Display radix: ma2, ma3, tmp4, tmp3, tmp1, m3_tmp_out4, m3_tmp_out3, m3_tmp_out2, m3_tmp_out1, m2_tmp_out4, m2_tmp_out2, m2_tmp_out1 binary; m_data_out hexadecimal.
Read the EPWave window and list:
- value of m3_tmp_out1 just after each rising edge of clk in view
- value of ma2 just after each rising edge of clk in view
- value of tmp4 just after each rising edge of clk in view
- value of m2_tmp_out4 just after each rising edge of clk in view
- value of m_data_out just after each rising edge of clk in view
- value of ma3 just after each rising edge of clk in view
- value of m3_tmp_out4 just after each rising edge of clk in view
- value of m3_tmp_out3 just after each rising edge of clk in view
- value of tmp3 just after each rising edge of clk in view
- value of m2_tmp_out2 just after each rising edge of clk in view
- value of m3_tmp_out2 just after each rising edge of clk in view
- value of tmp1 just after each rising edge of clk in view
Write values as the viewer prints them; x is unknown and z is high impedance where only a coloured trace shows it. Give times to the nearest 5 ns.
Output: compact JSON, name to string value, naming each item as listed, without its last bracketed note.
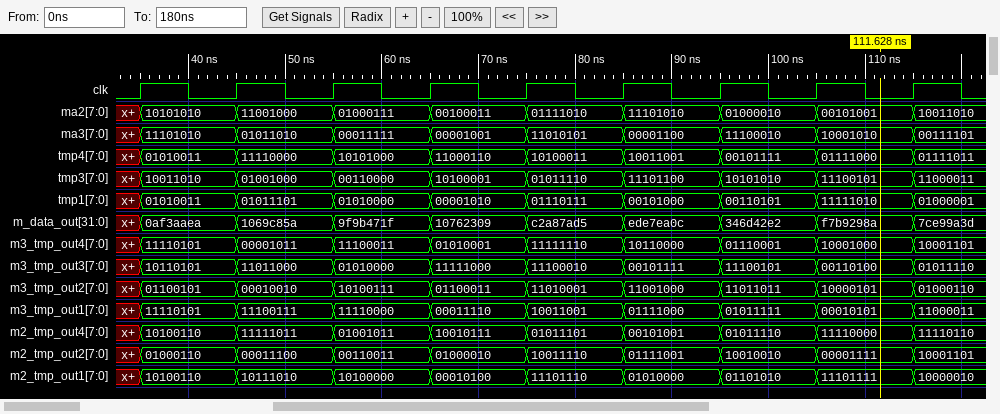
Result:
{"value of m3_tmp_out1 just after each rising edge of clk in view": "11110101, 11100111, 11110000, 00011110, 10011001, 01111000, 01011111, 00010101, 11000011", "value of ma2 just after each rising edge of clk in view": "10101010, 11001000, 01000111, 00100011, 01111010, 11101010, 01000010, 00101001, 10011010", "value of tmp4 just after each rising edge of clk in view": "01010011, 11110000, 10101000, 11000110, 10100011, 10011001, 00101111, 01111000, 01111011", "value of m2_tmp_out4 just after each rising edge of clk in view": "10100110, 11111011, 01001011, 10010111, 01011101, 00101001, 01011110, 11110000, 11110110", "value of m_data_out just after each rising edge of clk in view": "0af3aaea, 1069c85a, 9f9b471f, 10762309, c2a87ad5, ede7ea0c, 346d42e2, f7b9298a, 7ce99a3d", "value of ma3 just after each rising edge of clk in view": "11101010, 01011010, 00011111, 00001001, 11010101, 00001100, 11100010, 10001010, 00111101", "value of m3_tmp_out4 just after each rising edge of clk in view": "11110101, 00001011, 11100011, 01010001, 11111110, 10110000, 01110001, 10001000, 10001101", "value of m3_tmp_out3 just after each rising edge of clk in view": "10110101, 11011000, 01010000, 11111000, 11100010, 00101111, 11100101, 00110100, 01011110", "value of tmp3 just after each rising edge of clk in view": "10011010, 01001000, 00110000, 10100001, 01011110, 11101100, 10101010, 11100101, 11000011", "value of m2_tmp_out2 just after each rising edge of clk in view": "01000110, 00011100, 00110011, 01000010, 10011110, 01111001, 10010010, 00001111, 10001101", "value of m3_tmp_out2 just after each rising edge of clk in view": "01100101, 00010010, 10100111, 01100011, 11010001, 11001000, 11011011, 10000101, 01000110", "value of tmp1 just after each rising edge of clk in view": "01010011, 01011101, 01010000, 00001010, 01110111, 00101000, 00110101, 11111010, 01000001"}
